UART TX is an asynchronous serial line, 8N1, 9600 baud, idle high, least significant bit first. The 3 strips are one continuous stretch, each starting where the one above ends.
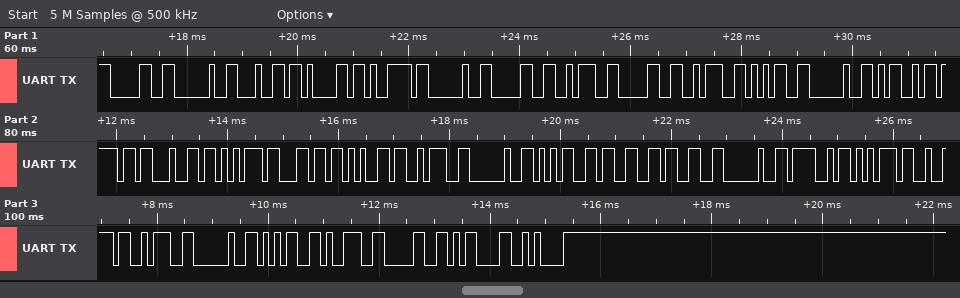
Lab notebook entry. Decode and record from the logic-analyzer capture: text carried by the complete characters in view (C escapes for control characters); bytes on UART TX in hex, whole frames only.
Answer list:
"0 day 0:0:5 Module: 533 Our: 590\r\n"
30 20 64 61 79 20 30 3A 30 3A 35 20 4D 6F 64 75 6C 65 3A 20 35 33 33 20 4F 75 72 3A 20 35 39 30 0D 0A
